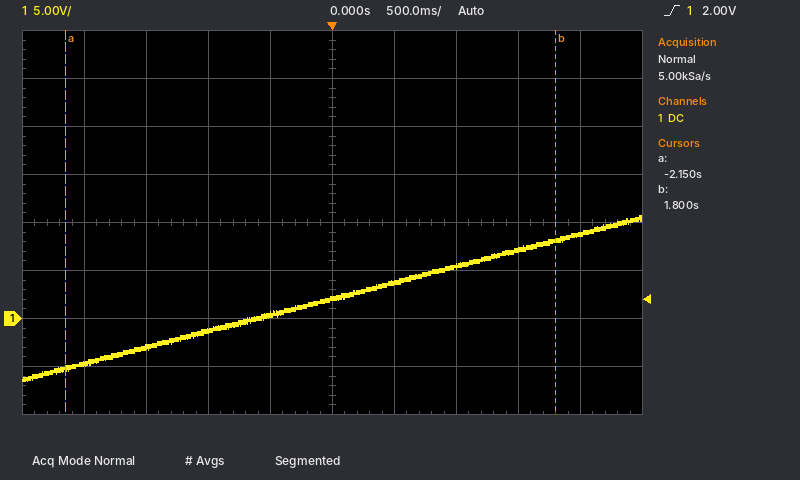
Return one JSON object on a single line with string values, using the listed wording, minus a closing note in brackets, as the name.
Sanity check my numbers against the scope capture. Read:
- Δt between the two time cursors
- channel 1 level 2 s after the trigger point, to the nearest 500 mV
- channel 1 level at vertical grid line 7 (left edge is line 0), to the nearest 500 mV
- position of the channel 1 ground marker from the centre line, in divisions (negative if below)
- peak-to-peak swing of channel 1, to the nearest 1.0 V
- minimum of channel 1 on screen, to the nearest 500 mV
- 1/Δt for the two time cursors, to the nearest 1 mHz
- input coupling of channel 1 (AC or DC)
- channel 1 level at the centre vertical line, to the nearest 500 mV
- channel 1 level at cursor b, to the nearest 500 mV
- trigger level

{"Δt between the two time cursors": "3.95 s", "channel 1 level 2 s after the trigger point, to the nearest 500 mV": "9.0 V", "channel 1 level at vertical grid line 7 (left edge is line 0), to the nearest 500 mV": "5.5 V", "position of the channel 1 ground marker from the centre line, in divisions": "-2.0 div", "peak-to-peak swing of channel 1, to the nearest 1.0 V": "17.0 V", "minimum of channel 1 on screen, to the nearest 500 mV": "-6.5 V", "1/Δt for the two time cursors, to the nearest 1 mHz": "253 mHz", "input coupling of channel 1": "DC", "channel 1 level at the centre vertical line, to the nearest 500 mV": "2.0 V", "channel 1 level at cursor b, to the nearest 500 mV": "8.0 V", "trigger level": "2.00 V"}
